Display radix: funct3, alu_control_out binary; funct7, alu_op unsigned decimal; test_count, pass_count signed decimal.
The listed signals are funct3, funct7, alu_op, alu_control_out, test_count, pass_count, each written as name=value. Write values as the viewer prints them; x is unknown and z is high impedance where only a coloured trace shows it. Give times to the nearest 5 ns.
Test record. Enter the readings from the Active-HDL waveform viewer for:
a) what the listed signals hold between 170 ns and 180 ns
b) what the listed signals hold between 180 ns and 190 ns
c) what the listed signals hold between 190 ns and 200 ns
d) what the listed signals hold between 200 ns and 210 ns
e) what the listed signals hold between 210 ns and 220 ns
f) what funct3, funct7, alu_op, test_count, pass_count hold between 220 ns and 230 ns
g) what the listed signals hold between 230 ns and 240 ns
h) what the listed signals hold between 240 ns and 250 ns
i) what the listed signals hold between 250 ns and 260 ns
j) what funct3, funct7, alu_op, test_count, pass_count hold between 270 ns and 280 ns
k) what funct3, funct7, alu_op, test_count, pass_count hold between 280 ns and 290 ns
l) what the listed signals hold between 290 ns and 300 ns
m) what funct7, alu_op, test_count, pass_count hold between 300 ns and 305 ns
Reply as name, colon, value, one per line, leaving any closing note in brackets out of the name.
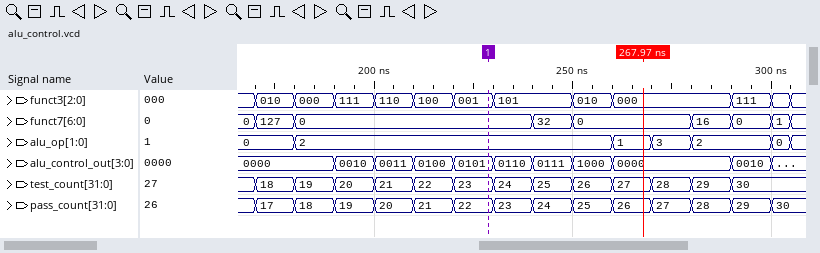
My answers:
what the listed signals hold between 170 ns and 180 ns: funct3=010, funct7=127, alu_op=0, alu_control_out=0000, test_count=18, pass_count=17
what the listed signals hold between 180 ns and 190 ns: funct3=000, funct7=0, alu_op=2, alu_control_out=0000, test_count=19, pass_count=18
what the listed signals hold between 190 ns and 200 ns: funct3=111, funct7=0, alu_op=2, alu_control_out=0010, test_count=20, pass_count=19
what the listed signals hold between 200 ns and 210 ns: funct3=110, funct7=0, alu_op=2, alu_control_out=0011, test_count=21, pass_count=20
what the listed signals hold between 210 ns and 220 ns: funct3=100, funct7=0, alu_op=2, alu_control_out=0100, test_count=22, pass_count=21
what funct3, funct7, alu_op, test_count, pass_count hold between 220 ns and 230 ns: funct3=001, funct7=0, alu_op=2, test_count=23, pass_count=22
what the listed signals hold between 230 ns and 240 ns: funct3=101, funct7=0, alu_op=2, alu_control_out=0110, test_count=24, pass_count=23
what the listed signals hold between 240 ns and 250 ns: funct3=101, funct7=32, alu_op=2, alu_control_out=0111, test_count=25, pass_count=24
what the listed signals hold between 250 ns and 260 ns: funct3=010, funct7=0, alu_op=2, alu_control_out=1000, test_count=26, pass_count=25
what funct3, funct7, alu_op, test_count, pass_count hold between 270 ns and 280 ns: funct3=000, funct7=0, alu_op=3, test_count=28, pass_count=27
what funct3, funct7, alu_op, test_count, pass_count hold between 280 ns and 290 ns: funct3=000, funct7=16, alu_op=2, test_count=29, pass_count=28
what the listed signals hold between 290 ns and 300 ns: funct3=111, funct7=0, alu_op=2, alu_control_out=0010, test_count=30, pass_count=29
what funct7, alu_op, test_count, pass_count hold between 300 ns and 305 ns: funct7=1, alu_op=0, test_count=30, pass_count=30
